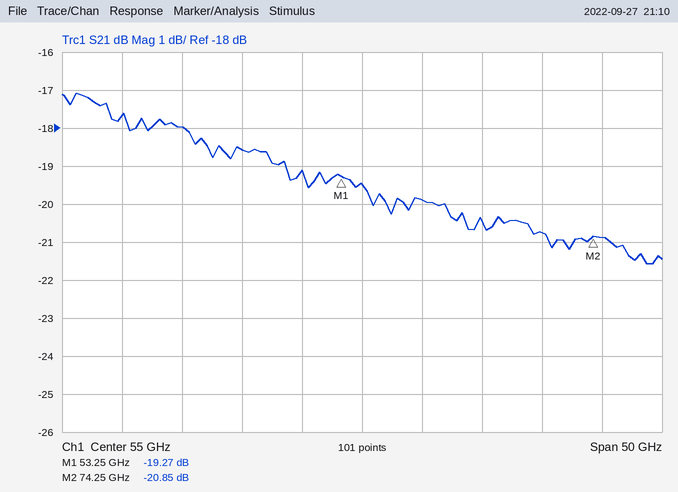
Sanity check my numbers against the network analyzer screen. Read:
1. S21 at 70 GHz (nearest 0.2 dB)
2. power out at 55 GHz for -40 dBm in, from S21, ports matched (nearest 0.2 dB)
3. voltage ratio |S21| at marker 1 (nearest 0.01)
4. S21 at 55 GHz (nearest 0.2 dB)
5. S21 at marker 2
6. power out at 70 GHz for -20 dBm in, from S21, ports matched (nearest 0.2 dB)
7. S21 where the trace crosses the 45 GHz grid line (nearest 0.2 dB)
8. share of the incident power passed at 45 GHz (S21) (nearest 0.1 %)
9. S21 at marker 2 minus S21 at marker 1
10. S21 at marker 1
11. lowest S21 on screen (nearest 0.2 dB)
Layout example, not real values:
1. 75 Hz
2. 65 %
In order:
1. -20.8 dB
2. -59.4 dBm
3. 0.11
4. -19.4 dB
5. -20.85 dB
6. -40.8 dBm
7. -18.6 dB
8. 1.4 %
9. -1.58 dB
10. -19.27 dB
11. -21.6 dB
